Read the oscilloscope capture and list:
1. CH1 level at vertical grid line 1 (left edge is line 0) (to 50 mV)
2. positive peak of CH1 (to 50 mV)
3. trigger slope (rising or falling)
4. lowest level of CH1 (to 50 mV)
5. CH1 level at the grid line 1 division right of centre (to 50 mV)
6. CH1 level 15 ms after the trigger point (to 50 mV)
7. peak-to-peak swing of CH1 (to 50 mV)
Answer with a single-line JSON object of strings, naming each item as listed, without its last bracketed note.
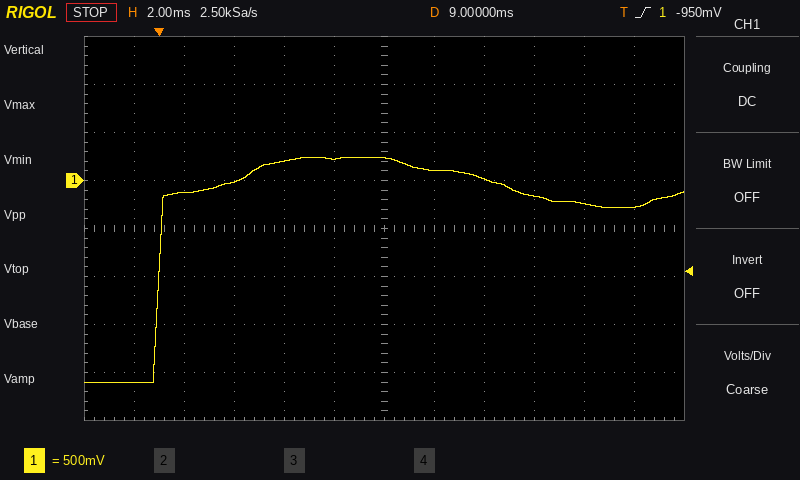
{"CH1 level at vertical grid line 1 (left edge is line 0)": "-2.10 V", "positive peak of CH1": "250 mV", "trigger slope": "rising", "lowest level of CH1": "-2.10 V", "CH1 level at the grid line 1 division right of centre": "100 mV", "CH1 level 15 ms after the trigger point": "-150 mV", "peak-to-peak swing of CH1": "2.35 V"}
